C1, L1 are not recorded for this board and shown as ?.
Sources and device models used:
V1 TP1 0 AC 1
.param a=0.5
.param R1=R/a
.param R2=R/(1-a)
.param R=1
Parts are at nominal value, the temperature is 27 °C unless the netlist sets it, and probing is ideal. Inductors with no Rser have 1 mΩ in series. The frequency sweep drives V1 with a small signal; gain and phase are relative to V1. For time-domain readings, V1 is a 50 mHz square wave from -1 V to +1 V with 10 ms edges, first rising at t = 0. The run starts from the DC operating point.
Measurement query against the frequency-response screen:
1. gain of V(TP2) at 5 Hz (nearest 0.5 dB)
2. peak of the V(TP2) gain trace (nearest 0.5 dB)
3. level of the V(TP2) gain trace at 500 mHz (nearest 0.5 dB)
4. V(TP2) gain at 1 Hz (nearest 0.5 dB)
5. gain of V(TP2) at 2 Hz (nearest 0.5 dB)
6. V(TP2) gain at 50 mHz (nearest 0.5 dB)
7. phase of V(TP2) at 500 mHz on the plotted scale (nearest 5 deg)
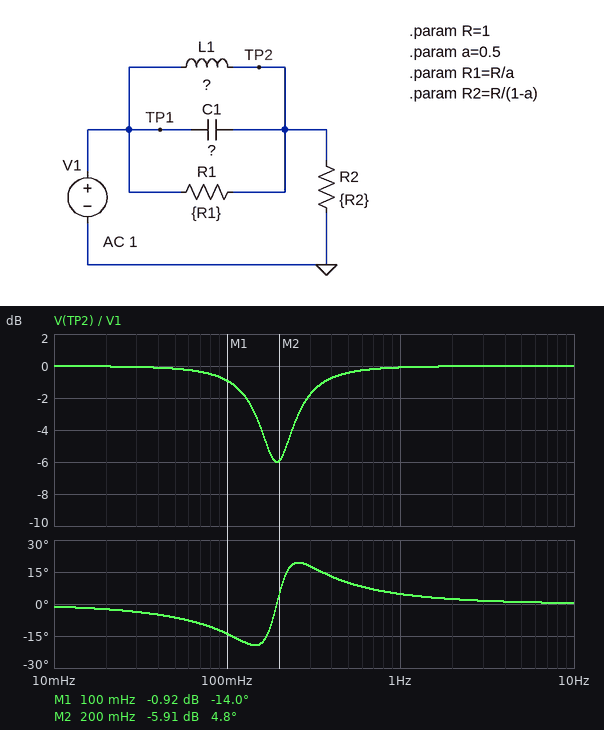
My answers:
0 dB
0 dB
-0.5 dB
0 dB
0 dB
0 dB
10 deg
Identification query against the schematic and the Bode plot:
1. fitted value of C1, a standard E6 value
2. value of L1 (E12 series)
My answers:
1 F
680 mH
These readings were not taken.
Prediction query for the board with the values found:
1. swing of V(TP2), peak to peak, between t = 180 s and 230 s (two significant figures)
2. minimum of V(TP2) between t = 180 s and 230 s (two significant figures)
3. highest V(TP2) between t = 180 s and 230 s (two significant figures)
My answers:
2.2 V
-1.1 V
1.1 V
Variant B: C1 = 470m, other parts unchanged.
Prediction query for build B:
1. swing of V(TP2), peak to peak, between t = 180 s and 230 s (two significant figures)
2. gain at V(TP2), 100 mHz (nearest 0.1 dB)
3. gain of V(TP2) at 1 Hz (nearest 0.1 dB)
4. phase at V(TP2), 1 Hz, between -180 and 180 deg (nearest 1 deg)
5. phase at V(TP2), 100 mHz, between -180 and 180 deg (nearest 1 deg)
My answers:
2.1 V
-0.7 dB
-0.4 dB
10 deg
-12 deg
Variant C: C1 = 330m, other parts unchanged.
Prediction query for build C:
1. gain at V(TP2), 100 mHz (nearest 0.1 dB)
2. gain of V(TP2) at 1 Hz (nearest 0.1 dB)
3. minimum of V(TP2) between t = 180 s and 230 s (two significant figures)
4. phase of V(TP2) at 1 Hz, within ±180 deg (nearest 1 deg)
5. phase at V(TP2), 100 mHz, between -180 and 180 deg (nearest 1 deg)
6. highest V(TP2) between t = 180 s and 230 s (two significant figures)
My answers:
-0.6 dB
-0.8 dB
-1.0 V
13 deg
-12 deg
1.0 V
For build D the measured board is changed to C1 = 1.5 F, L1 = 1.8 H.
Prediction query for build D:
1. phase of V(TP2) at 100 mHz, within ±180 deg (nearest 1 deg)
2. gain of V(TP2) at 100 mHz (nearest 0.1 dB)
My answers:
3 deg
-6.0 dB
